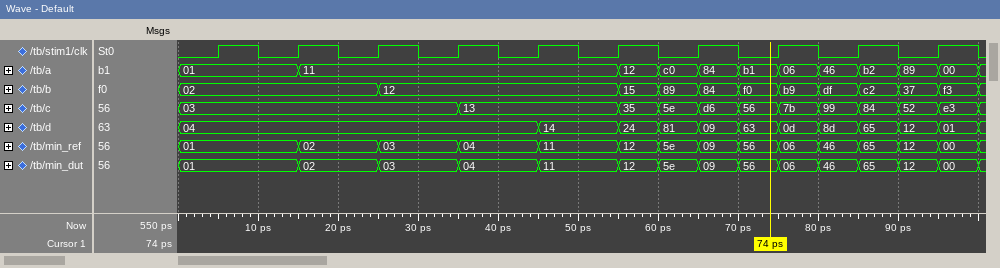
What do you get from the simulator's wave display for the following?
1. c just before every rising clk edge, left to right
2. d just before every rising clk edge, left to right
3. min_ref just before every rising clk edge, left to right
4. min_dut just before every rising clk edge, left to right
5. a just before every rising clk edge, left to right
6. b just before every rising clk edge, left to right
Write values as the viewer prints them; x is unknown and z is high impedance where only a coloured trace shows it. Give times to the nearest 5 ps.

03, 03, 03, 03, 13, 13, 5e, 56, 99, 52
04, 04, 04, 04, 04, 14, 81, 63, 8d, 12
01, 01, 02, 03, 04, 11, 5e, 56, 46, 12
01, 01, 02, 03, 04, 11, 5e, 56, 46, 12
01, 01, 11, 11, 11, 11, c0, b1, 46, 89
02, 02, 02, 12, 12, 12, 89, f0, df, 37
